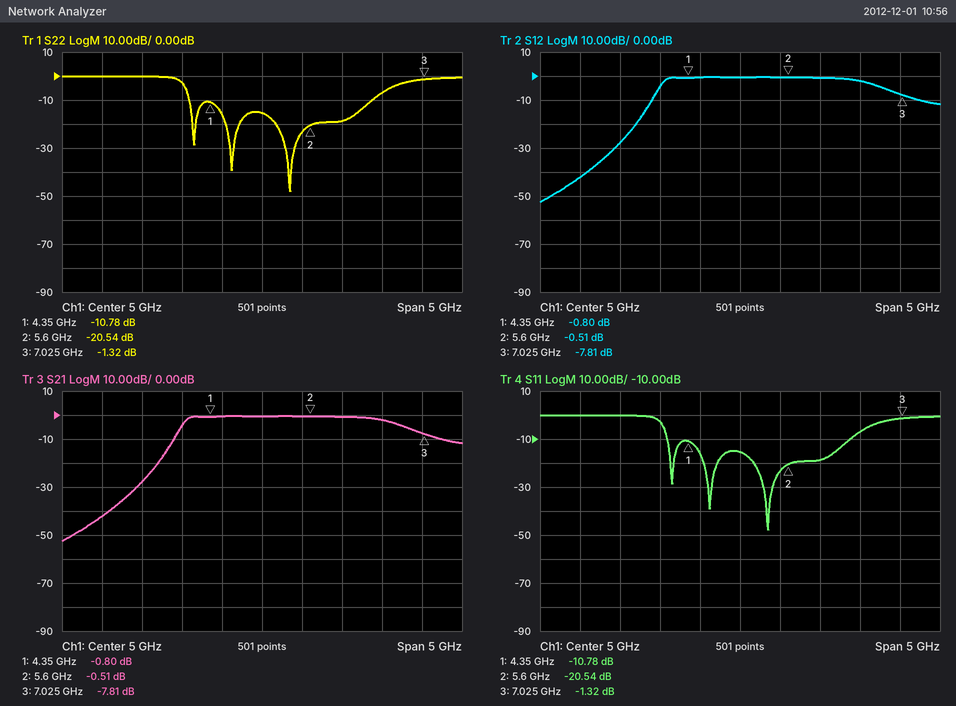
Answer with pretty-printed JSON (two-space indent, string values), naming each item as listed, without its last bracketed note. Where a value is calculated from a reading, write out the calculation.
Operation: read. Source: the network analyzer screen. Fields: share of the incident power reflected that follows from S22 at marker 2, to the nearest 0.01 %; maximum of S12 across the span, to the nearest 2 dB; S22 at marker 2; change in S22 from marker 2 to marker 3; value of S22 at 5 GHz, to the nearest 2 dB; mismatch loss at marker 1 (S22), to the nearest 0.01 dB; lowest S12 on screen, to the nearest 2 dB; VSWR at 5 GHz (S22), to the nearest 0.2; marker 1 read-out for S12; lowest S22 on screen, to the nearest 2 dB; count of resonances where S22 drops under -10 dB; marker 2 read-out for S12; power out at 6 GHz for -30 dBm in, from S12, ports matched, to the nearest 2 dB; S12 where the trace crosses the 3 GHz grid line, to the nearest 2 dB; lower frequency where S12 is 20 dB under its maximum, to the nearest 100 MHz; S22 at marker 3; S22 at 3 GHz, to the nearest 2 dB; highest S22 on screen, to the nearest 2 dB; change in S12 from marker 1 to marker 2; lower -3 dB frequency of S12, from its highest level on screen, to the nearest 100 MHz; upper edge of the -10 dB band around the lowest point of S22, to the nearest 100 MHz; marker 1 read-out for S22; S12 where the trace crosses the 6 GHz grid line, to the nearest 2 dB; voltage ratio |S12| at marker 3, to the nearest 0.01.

{
  "share of the incident power reflected that follows from S22 at marker 2, to the nearest 0.01 %": "10^(-20.54/10) ≈ 0.88 %",
  "maximum of S12 across the span, to the nearest 2 dB": "0 dB",
  "S22 at marker 2": "-20.54 dB",
  "change in S22 from marker 2 to marker 3": "-1.32 − (-20.54) = 19.22 dB",
  "value of S22 at 5 GHz, to the nearest 2 dB": "-16 dB",
  "mismatch loss at marker 1 (S22), to the nearest 0.01 dB": "−10 log10(1 − 10^(-10.78/10)) ≈ 0.38 dB",
  "lowest S12 on screen, to the nearest 2 dB": "-52 dB",
  "VSWR at 5 GHz (S22), to the nearest 0.2": "|Γ| = 10^(-16/20) = 0.1585; VSWR = (1 + 0.1585)/(1 − 0.1585) ≈ 1.4",
  "marker 1 read-out for S12": "-0.80 dB",
  "lowest S22 on screen, to the nearest 2 dB": "-48 dB",
  "count of resonances where S22 drops under -10 dB": "3",
  "marker 2 read-out for S12": "-0.51 dB",
  "power out at 6 GHz for -30 dBm in, from S12, ports matched, to the nearest 2 dB": "-30 dBm + (0 dB) = -30 dBm",
  "S12 where the trace crosses the 3 GHz grid line, to the nearest 2 dB": "-42 dB",
  "lower frequency where S12 is 20 dB under its maximum, to the nearest 100 MHz": "3.7 GHz",
  "S22 at marker 3": "-1.32 dB",
  "S22 at 3 GHz, to the nearest 2 dB": "0 dB",
  "highest S22 on screen, to the nearest 2 dB": "0 dB",
  "change in S12 from marker 1 to marker 2": "-0.51 − (-0.8) = 0.29 dB",
  "lower -3 dB frequency of S12, from its highest level on screen, to the nearest 100 MHz": "4.0 GHz",
  "upper edge of the -10 dB band around the lowest point of S22, to the nearest 100 MHz": "6.4 GHz",
  "marker 1 read-out for S22": "-10.78 dB",
  "S12 where the trace crosses the 6 GHz grid line, to the nearest 2 dB": "0 dB",
  "voltage ratio |S12| at marker 3, to the nearest 0.01": "10^(-7.81/20) ≈ 0.41"
}
